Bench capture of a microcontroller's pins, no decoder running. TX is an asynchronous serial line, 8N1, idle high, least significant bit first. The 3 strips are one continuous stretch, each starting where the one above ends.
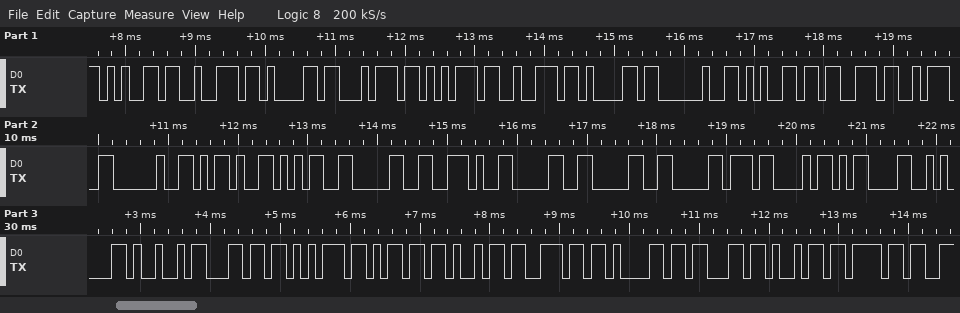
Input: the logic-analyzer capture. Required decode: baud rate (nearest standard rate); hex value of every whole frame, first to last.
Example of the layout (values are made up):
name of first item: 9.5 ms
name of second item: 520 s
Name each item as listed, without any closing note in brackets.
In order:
baud rate: 9600 baud
hex value of every whole frame, first to last: 65 72 61 74 75 72 61 20 65 73 3A 20 2D 35 30 2E 30 30 B0 43 0D 0A 49 6C 75 6D 69 6E 61 63 69 6F
